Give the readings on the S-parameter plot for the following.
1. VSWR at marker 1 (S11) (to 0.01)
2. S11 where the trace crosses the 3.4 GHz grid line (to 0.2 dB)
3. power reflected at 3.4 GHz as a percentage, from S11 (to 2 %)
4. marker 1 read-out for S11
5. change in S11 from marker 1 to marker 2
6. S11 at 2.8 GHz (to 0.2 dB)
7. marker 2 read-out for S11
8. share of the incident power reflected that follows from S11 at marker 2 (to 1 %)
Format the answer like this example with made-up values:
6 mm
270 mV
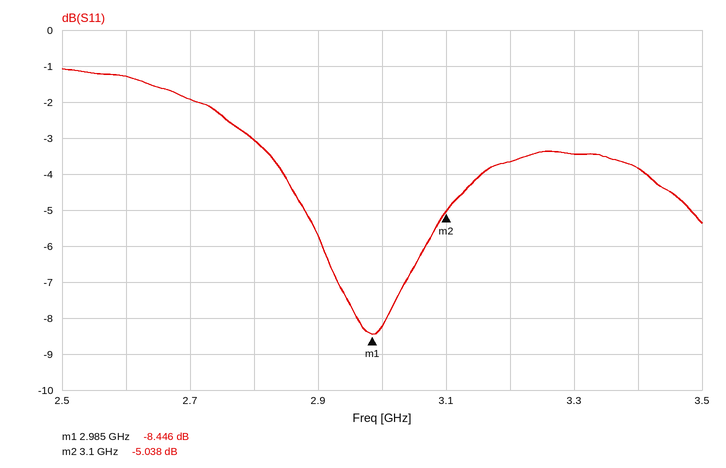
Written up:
2.22
-3.8 dB
42 %
-8.446 dB
3.408 dB
-3.0 dB
-5.038 dB
31 %
